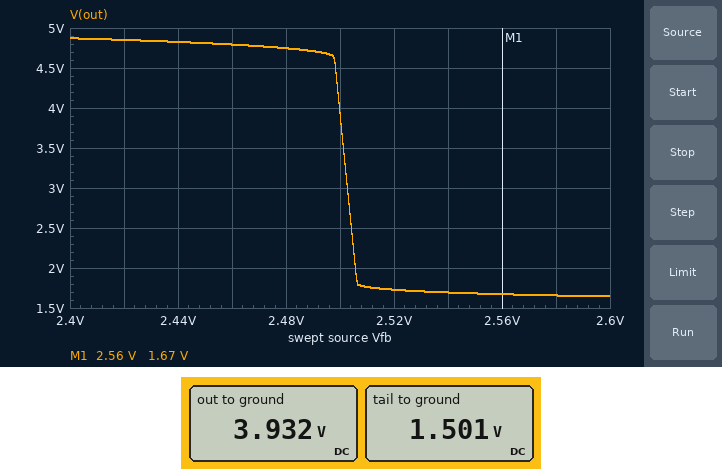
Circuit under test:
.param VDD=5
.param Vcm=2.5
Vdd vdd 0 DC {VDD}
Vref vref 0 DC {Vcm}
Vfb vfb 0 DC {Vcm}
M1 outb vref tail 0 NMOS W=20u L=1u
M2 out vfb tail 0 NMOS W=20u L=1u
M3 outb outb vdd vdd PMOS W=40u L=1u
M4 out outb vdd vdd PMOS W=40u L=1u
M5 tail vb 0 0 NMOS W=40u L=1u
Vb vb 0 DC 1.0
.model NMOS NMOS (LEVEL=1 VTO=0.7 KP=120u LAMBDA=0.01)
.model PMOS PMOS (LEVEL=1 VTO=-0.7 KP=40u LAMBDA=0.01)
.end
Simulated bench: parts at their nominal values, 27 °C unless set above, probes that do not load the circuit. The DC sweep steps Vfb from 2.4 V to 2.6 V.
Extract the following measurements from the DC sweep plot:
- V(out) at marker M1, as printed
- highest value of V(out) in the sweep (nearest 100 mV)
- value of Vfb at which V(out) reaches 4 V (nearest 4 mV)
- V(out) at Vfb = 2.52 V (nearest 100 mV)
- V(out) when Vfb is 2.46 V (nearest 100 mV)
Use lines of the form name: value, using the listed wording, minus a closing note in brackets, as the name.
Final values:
V(out) at marker M1, as printed: 1.67 V
highest value of V(out) in the sweep: 4.9 V
value of Vfb at which V(out) reaches 4 V: 2.500 V
V(out) at Vfb = 2.52 V: 1.7 V
V(out) when Vfb is 2.46 V: 4.8 V
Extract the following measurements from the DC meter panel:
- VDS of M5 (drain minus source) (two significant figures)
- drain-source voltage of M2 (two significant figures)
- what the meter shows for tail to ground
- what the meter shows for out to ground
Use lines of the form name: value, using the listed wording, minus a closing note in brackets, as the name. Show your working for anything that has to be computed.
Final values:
VDS of M5 (drain minus source): 1.501 V = 1.5 V
drain-source voltage of M2: 3.932 V - 1.501 V = 2.4 V
what the meter shows for tail to ground: 1.501 V
what the meter shows for out to ground: 3.932 V
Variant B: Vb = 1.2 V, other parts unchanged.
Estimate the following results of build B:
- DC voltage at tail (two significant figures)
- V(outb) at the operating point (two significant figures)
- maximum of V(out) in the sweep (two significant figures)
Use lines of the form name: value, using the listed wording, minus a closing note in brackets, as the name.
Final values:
DC voltage at tail: 1.3 V
V(outb) at the operating point: 3.7 V
maximum of V(out) in the sweep: 4.7 V
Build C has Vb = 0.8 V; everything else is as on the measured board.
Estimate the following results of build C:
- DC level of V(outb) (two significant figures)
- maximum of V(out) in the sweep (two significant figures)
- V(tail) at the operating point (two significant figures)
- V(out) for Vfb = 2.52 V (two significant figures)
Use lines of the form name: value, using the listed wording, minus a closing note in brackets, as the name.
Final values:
DC level of V(outb): 4.2 V
maximum of V(out) in the sweep: 5.0 V
V(tail) at the operating point: 1.7 V
V(out) for Vfb = 2.52 V: 1.8 V
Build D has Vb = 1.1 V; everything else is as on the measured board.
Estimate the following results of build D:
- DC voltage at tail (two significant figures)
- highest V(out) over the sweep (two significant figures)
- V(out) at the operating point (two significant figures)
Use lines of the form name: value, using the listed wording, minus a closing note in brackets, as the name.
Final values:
DC voltage at tail: 1.4 V
highest V(out) over the sweep: 4.8 V
V(out) at the operating point: 3.8 V
